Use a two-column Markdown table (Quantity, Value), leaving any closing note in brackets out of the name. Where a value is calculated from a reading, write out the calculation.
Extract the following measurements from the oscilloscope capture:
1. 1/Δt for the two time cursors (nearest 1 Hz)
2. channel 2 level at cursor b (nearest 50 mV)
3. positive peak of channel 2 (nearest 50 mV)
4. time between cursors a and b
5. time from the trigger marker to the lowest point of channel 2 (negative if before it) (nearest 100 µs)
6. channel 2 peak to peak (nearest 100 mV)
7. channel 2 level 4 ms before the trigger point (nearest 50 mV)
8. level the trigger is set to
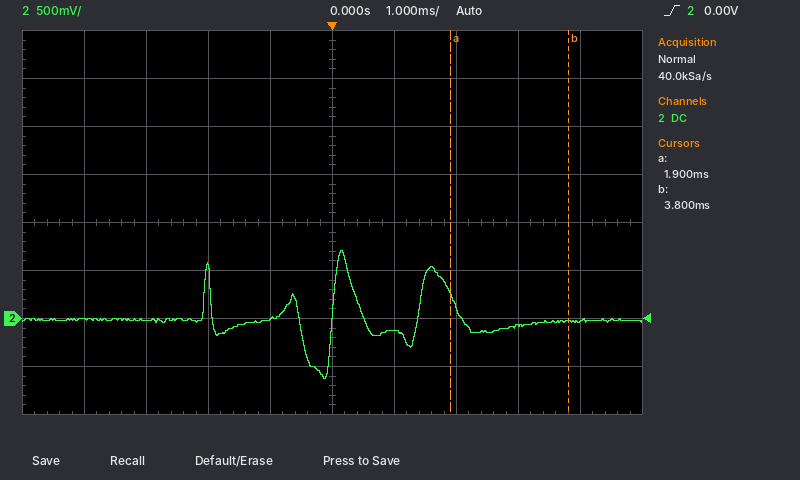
| Quantity | Value |
|---|---|
| 1/Δt for the two time cursors | 1 / 1.9 ms ≈ 526 Hz |
| channel 2 level at cursor b | -50 mV |
| positive peak of channel 2 | 700 mV |
| time between cursors a and b | 3.8 ms − (1.9 ms) = 1.9 ms |
| time from the trigger marker to the lowest point of channel 2 (negative if before it) | -100 µs |
| channel 2 peak to peak | 1.30 V |
| channel 2 level 4 ms before the trigger point | 0 mV |
| level the trigger is set to | 0.00 V |
